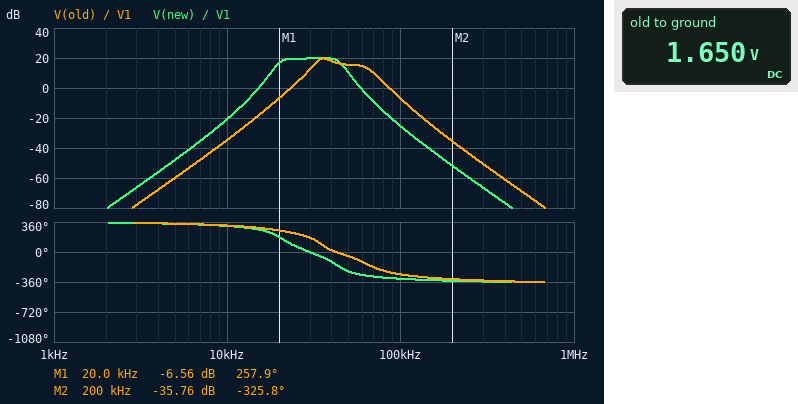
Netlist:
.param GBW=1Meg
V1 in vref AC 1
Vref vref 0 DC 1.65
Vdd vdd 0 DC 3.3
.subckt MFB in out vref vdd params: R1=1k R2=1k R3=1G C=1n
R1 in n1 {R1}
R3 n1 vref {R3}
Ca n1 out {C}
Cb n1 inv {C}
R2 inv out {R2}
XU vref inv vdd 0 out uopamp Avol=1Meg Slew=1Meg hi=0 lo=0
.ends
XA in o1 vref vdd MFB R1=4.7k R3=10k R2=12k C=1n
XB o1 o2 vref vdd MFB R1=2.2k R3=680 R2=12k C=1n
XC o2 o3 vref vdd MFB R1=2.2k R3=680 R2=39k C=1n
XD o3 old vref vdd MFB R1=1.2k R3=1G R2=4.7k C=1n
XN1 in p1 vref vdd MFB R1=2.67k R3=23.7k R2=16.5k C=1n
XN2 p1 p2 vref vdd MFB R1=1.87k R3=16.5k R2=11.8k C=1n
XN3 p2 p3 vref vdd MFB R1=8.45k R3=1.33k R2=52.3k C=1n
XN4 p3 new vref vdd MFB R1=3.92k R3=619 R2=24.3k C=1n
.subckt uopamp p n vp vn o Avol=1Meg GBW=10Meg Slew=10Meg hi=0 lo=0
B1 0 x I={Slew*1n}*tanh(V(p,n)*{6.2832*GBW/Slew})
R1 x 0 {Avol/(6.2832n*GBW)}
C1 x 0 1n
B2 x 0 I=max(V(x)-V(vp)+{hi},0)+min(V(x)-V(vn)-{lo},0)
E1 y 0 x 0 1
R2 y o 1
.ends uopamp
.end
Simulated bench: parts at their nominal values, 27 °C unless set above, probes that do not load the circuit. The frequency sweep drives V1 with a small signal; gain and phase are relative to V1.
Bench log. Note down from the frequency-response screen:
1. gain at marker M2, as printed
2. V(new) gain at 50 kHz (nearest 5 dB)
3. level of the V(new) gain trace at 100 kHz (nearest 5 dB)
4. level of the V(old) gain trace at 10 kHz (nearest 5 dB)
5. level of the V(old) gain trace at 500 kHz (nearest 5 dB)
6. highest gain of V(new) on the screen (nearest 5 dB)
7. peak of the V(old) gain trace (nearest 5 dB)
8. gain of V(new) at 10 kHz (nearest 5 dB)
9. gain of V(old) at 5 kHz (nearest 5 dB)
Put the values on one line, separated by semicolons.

-35.76 dB; 10 dB; -25 dB; -35 dB; -70 dB; 20 dB; 20 dB; -20 dB; -60 dB
